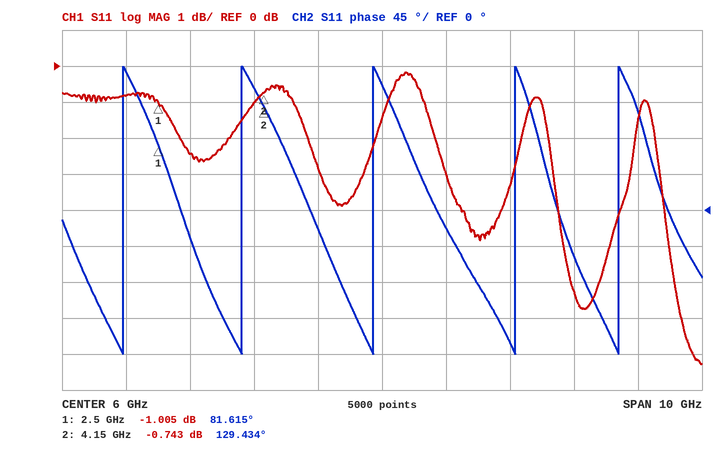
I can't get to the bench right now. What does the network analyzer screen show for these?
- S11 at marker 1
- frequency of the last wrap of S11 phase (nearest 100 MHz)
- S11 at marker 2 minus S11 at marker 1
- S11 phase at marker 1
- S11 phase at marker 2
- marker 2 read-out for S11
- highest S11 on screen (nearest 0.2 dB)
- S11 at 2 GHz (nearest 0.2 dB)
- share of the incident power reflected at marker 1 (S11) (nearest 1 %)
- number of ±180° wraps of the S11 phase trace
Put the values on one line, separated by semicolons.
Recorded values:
-1.005 dB; 9.7 GHz; 0.262 dB; 81.615°; 129.434°; -0.743 dB; -0.2 dB; -0.8 dB; 79 %; 5
